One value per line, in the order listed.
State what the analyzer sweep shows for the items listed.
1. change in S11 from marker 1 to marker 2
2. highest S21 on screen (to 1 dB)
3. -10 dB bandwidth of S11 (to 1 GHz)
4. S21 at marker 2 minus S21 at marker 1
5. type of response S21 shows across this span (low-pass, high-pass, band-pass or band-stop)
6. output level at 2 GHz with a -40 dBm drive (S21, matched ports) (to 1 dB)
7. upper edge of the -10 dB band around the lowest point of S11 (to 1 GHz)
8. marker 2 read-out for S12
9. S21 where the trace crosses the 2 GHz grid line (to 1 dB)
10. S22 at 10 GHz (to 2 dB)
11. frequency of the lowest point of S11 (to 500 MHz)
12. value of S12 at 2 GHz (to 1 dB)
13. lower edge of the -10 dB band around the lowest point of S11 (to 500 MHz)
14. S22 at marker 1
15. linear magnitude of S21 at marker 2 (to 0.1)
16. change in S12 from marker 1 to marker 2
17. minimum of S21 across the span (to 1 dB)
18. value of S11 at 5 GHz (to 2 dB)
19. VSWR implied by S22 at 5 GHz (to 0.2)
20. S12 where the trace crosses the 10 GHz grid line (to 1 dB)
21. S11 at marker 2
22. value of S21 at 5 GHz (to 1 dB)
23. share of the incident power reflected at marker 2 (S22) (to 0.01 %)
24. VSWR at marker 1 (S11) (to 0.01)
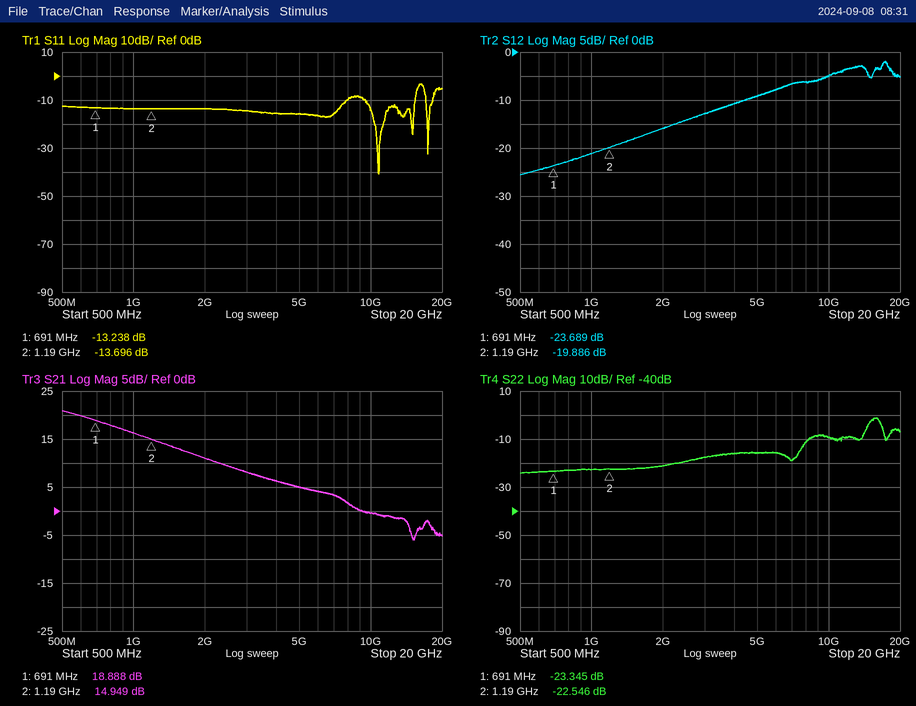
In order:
-0.458 dB
21 dB
6 GHz
-3.939 dB
low-pass
-29 dBm
15 GHz
-19.886 dB
11 dB
-10 dB
11.0 GHz
-16 dB
9.5 GHz
-23.345 dB
5.6
3.803 dB
-6 dB
-16 dB
1.4
-5 dB
-13.696 dB
5 dB
0.56 %
1.56
